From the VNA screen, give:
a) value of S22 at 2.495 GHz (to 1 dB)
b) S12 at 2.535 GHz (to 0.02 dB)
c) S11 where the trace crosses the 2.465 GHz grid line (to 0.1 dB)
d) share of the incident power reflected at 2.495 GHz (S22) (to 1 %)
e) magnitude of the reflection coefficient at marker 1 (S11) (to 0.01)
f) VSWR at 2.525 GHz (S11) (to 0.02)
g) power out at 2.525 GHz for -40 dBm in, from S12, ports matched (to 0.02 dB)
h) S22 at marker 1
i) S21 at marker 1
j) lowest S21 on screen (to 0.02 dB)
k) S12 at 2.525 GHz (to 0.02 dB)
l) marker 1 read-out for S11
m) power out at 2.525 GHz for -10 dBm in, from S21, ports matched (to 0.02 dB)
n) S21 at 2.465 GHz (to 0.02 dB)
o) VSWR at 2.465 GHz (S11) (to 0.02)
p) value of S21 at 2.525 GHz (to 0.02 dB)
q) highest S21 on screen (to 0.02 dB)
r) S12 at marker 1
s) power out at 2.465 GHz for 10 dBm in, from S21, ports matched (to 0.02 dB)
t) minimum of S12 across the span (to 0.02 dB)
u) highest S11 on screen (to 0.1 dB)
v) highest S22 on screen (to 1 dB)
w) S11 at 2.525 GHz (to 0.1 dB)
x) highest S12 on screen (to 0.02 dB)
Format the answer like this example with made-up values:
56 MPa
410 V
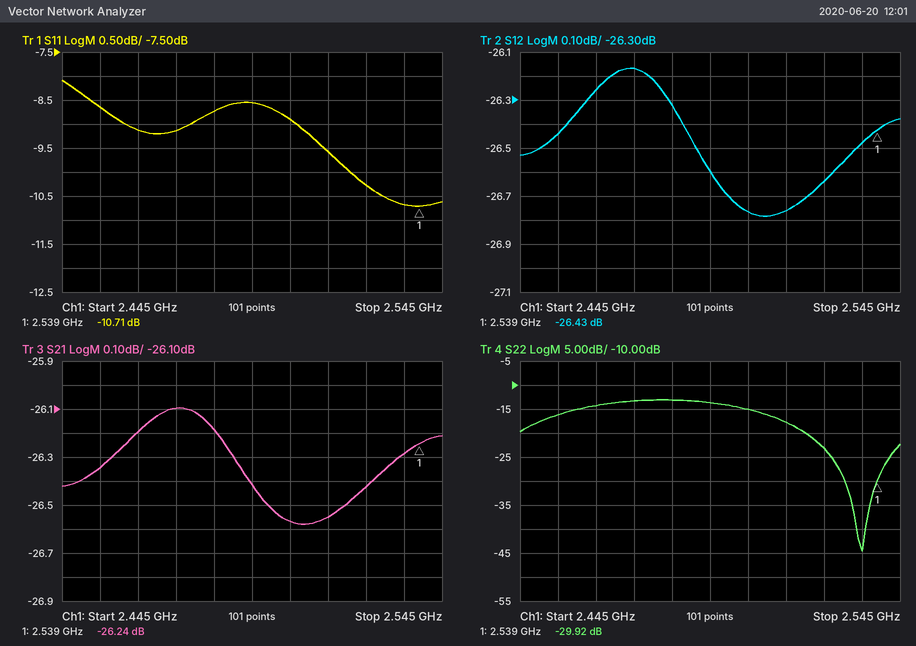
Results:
-14 dB
-26.48 dB
-9.1 dB
4 %
0.29
1.88
-66.64 dBm
-29.92 dB
-26.24 dB
-26.58 dB
-26.64 dB
-10.71 dB
-36.42 dBm
-26.20 dB
2.08
-26.42 dB
-26.10 dB
-26.43 dB
-16.20 dBm
-26.78 dB
-8.1 dB
-13 dB
-10.3 dB
-26.16 dB
